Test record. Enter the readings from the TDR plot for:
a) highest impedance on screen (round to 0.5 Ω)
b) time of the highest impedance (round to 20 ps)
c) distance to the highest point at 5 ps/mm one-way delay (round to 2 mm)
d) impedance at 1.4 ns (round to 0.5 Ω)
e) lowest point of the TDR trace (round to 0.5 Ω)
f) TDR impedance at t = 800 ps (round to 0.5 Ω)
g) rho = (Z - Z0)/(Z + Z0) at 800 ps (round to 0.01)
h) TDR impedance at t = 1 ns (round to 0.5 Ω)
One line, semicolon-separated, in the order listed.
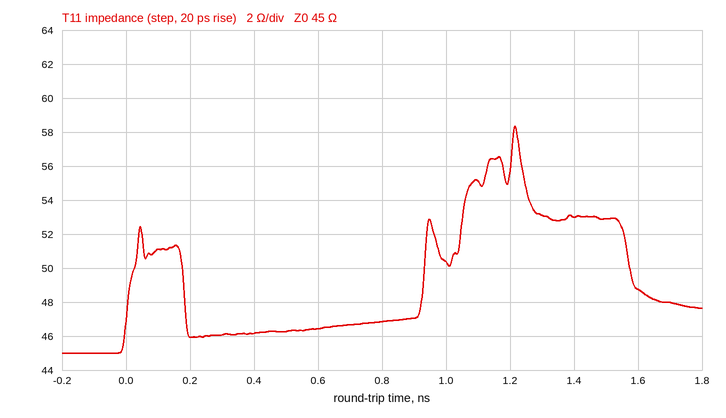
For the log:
58.5 Ω; 1.22 ns; 122 mm; 53.0 Ω; 45.0 Ω; 47.0 Ω; +0.02; 50.5 Ω
